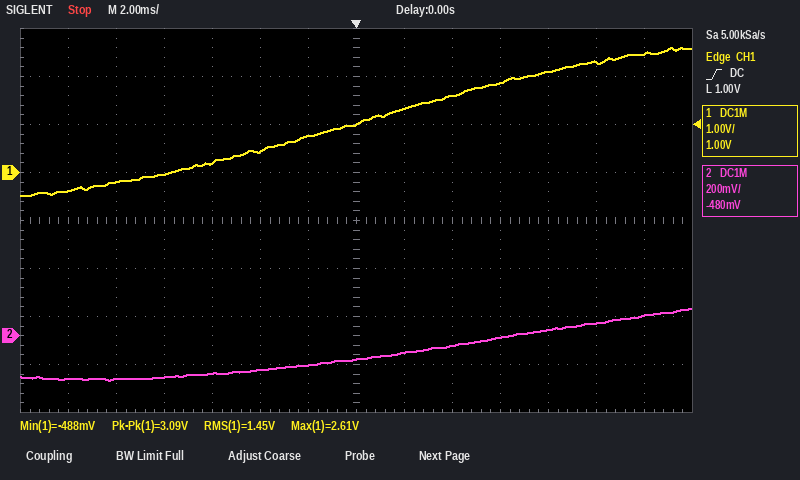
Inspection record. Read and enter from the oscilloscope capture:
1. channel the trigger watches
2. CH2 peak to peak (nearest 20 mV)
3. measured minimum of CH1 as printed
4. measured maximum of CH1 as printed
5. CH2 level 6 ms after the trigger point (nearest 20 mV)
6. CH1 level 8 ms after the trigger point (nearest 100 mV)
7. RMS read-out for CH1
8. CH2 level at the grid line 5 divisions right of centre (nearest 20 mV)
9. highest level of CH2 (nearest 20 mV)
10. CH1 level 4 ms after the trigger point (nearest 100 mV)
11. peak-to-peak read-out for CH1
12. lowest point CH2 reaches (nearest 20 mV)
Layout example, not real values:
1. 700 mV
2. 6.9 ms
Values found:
1. CH1
2. 300 mV
3. -488 mV
4. 2.61 V
5. 0 mV
6. 2.1 V
7. 1.45 V
8. 60 mV
9. 120 mV
10. 1.6 V
11. 3.09 V
12. -180 mV
